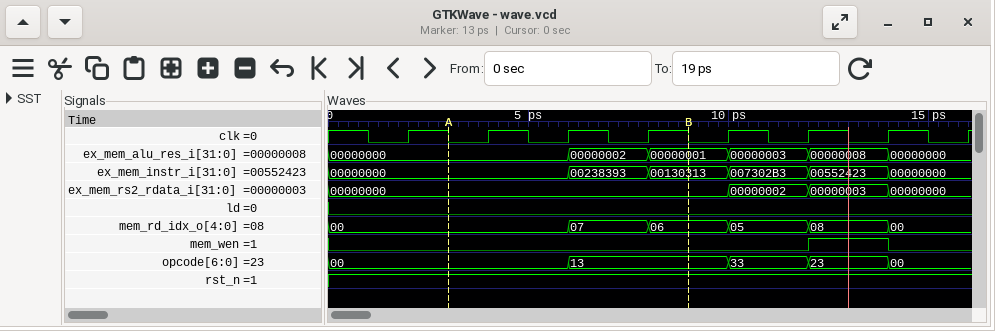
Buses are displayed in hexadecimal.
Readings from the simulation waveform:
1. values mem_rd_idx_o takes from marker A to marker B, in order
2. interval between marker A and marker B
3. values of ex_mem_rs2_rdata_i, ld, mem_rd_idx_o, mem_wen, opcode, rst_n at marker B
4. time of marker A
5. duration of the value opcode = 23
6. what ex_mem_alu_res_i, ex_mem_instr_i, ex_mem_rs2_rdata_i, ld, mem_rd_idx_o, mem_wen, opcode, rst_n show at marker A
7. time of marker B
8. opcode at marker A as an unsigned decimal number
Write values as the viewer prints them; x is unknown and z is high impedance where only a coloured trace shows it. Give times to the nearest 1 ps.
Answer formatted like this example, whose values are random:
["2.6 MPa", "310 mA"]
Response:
["00, 07, 06", "6 ps", "ex_mem_rs2_rdata_i=00000000, ld=0, mem_rd_idx_o=06, mem_wen=0, opcode=13, rst_n=1", "3 ps", "2 ps", "ex_mem_alu_res_i=00000000, ex_mem_instr_i=00000000, ex_mem_rs2_rdata_i=00000000, ld=0, mem_rd_idx_o=00, mem_wen=0, opcode=00, rst_n=1", "9 ps", "0"]
